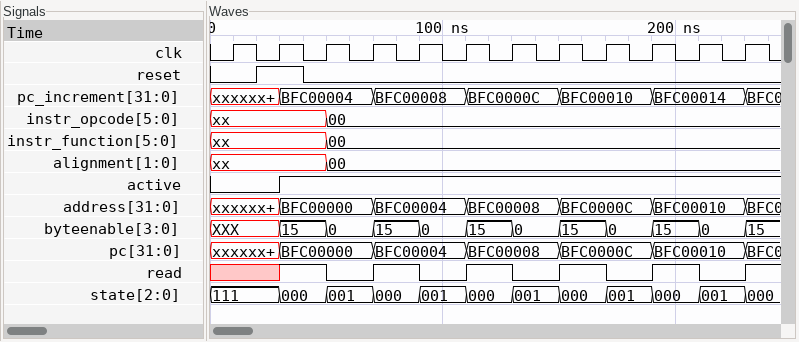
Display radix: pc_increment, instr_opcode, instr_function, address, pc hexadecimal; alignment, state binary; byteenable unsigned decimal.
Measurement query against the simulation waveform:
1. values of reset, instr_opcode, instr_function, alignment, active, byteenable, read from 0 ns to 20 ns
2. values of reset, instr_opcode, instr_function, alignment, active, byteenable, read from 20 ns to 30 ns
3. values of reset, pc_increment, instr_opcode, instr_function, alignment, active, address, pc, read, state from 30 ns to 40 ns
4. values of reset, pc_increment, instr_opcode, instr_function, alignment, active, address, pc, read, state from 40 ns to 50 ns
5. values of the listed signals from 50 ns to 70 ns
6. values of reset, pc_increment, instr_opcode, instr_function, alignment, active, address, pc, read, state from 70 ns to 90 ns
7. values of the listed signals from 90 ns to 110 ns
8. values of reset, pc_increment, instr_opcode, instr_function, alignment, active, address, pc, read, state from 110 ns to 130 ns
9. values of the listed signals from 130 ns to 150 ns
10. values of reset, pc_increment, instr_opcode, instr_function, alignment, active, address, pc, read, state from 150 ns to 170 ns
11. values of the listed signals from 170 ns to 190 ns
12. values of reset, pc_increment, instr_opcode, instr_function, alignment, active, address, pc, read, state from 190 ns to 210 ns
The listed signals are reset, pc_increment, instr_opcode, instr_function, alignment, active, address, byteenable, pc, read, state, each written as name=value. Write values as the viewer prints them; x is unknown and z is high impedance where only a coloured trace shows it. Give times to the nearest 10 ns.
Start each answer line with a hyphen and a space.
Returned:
- reset=0, instr_opcode=xx, instr_function=xx, alignment=xx, active=0, byteenable=XXX, read=x
- reset=1, instr_opcode=xx, instr_function=xx, alignment=xx, active=0, byteenable=XXX, read=x
- reset=1, pc_increment=BFC00004, instr_opcode=xx, instr_function=xx, alignment=xx, active=1, address=BFC00000, pc=BFC00000, read=1, state=000
- reset=0, pc_increment=BFC00004, instr_opcode=xx, instr_function=xx, alignment=xx, active=1, address=BFC00000, pc=BFC00000, read=1, state=000
- reset=0, pc_increment=BFC00004, instr_opcode=00, instr_function=00, alignment=00, active=1, address=BFC00000, byteenable=0, pc=BFC00000, read=0, state=001
- reset=0, pc_increment=BFC00008, instr_opcode=00, instr_function=00, alignment=00, active=1, address=BFC00004, pc=BFC00004, read=1, state=000
- reset=0, pc_increment=BFC00008, instr_opcode=00, instr_function=00, alignment=00, active=1, address=BFC00004, byteenable=0, pc=BFC00004, read=0, state=001
- reset=0, pc_increment=BFC0000C, instr_opcode=00, instr_function=00, alignment=00, active=1, address=BFC00008, pc=BFC00008, read=1, state=000
- reset=0, pc_increment=BFC0000C, instr_opcode=00, instr_function=00, alignment=00, active=1, address=BFC00008, byteenable=0, pc=BFC00008, read=0, state=001
- reset=0, pc_increment=BFC00010, instr_opcode=00, instr_function=00, alignment=00, active=1, address=BFC0000C, pc=BFC0000C, read=1, state=000
- reset=0, pc_increment=BFC00010, instr_opcode=00, instr_function=00, alignment=00, active=1, address=BFC0000C, byteenable=0, pc=BFC0000C, read=0, state=001
- reset=0, pc_increment=BFC00014, instr_opcode=00, instr_function=00, alignment=00, active=1, address=BFC00010, pc=BFC00010, read=1, state=000
